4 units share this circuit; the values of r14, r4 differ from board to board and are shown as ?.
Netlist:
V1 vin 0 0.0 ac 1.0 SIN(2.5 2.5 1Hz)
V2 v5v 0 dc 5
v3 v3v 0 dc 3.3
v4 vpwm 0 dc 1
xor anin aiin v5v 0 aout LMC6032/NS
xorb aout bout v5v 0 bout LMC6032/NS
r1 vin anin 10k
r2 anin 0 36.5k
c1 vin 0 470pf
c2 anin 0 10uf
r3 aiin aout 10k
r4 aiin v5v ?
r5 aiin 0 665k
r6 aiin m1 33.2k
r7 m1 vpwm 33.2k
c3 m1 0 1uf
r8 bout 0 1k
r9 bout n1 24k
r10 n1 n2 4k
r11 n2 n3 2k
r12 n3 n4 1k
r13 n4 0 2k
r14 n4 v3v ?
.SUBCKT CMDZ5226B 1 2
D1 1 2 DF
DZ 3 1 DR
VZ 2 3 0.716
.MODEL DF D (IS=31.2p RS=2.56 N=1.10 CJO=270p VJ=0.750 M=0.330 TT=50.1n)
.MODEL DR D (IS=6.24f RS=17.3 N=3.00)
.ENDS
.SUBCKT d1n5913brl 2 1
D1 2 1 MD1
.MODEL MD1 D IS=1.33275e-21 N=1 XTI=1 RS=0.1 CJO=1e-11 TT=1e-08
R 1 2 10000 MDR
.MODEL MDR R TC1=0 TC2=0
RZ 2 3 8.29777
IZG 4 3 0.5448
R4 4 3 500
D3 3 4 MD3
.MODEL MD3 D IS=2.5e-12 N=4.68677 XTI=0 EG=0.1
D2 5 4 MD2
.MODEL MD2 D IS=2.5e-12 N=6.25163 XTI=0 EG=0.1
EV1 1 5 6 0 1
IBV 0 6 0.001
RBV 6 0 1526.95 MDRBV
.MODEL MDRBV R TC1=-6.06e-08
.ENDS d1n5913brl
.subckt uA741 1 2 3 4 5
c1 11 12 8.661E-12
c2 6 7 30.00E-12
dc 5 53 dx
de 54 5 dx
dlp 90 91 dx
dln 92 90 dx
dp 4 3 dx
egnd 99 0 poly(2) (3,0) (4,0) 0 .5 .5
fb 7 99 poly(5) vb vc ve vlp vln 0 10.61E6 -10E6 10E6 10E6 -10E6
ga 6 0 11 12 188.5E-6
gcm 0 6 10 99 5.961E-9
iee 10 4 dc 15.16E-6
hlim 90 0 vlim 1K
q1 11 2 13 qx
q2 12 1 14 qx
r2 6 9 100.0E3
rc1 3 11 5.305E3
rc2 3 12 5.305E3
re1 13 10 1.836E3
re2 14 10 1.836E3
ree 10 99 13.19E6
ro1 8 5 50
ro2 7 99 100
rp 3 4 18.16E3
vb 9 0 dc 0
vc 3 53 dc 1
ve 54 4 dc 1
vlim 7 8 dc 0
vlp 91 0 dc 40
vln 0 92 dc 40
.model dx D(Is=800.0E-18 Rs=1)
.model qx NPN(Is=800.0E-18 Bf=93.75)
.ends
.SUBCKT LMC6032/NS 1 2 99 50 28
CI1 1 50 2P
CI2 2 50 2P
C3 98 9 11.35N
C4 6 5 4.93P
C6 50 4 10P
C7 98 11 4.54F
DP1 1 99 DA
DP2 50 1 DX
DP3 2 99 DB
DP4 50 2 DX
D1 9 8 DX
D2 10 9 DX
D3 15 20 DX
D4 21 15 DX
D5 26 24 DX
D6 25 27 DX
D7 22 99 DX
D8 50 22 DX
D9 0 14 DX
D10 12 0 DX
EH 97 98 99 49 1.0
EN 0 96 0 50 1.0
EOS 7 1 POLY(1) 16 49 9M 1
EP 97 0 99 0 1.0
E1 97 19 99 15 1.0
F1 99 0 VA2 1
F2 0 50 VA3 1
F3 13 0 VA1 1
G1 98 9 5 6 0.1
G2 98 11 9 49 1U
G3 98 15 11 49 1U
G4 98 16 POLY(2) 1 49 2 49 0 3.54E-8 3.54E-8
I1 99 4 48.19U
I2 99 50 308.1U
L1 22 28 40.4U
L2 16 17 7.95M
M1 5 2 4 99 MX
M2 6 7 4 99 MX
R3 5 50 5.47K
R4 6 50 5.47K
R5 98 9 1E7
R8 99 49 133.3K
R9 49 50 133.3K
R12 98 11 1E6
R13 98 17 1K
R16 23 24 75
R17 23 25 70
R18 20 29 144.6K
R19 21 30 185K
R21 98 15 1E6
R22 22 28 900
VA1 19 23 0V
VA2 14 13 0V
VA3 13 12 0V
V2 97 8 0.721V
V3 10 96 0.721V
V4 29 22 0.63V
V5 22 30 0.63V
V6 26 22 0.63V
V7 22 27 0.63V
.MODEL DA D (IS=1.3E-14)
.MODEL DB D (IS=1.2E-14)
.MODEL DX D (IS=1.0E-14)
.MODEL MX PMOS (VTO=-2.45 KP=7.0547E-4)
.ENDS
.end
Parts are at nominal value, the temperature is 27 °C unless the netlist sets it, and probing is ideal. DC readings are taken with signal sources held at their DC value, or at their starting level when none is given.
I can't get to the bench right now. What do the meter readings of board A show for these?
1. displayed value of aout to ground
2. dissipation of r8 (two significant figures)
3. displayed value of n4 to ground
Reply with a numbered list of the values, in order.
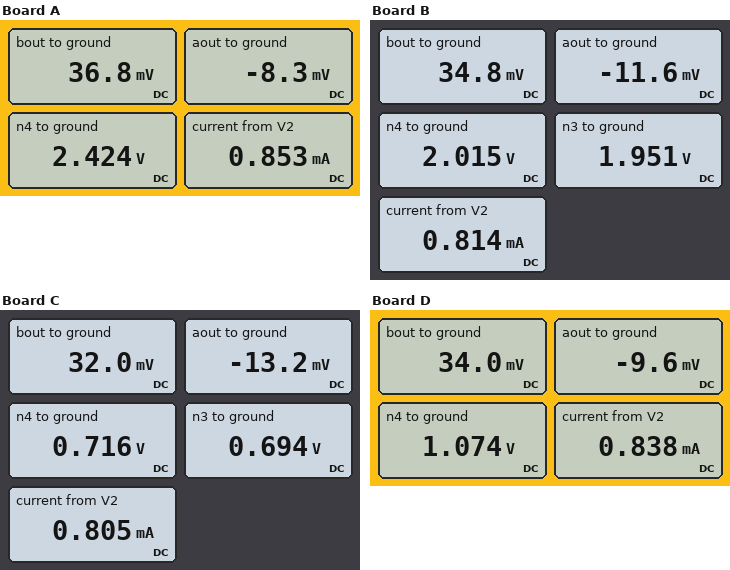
1. -8.3 mV
2. 1.4 µW
3. 2.424 V
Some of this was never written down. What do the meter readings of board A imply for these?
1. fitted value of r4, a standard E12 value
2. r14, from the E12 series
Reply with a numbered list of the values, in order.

1. 39 kΩ
2. 680 Ω
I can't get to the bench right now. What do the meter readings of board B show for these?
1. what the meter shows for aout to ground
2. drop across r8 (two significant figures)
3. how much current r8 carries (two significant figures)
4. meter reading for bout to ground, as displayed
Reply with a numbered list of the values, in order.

1. -11.6 mV
2. 35 mV
3. 35 µA
4. 34.8 mV
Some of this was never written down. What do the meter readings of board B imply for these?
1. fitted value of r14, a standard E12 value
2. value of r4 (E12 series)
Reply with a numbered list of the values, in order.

1. 1.2 kΩ
2. 68 kΩ
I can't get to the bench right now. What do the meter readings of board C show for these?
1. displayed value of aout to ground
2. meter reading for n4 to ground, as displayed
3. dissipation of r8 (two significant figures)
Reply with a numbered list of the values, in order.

1. -13.2 mV
2. 0.716 V
3. 1.0 µW
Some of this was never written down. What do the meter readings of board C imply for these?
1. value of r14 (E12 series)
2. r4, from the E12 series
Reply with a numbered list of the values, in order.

1. 6.8 kΩ
2. 100 kΩ
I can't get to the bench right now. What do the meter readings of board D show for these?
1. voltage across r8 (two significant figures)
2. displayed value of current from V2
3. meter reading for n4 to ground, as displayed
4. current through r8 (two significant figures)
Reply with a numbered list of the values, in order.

1. 34 mV
2. 0.838 mA
3. 1.074 V
4. 34 µA
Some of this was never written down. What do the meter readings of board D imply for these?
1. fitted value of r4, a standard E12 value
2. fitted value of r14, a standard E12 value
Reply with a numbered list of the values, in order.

1. 47 kΩ
2. 3.9 kΩ
